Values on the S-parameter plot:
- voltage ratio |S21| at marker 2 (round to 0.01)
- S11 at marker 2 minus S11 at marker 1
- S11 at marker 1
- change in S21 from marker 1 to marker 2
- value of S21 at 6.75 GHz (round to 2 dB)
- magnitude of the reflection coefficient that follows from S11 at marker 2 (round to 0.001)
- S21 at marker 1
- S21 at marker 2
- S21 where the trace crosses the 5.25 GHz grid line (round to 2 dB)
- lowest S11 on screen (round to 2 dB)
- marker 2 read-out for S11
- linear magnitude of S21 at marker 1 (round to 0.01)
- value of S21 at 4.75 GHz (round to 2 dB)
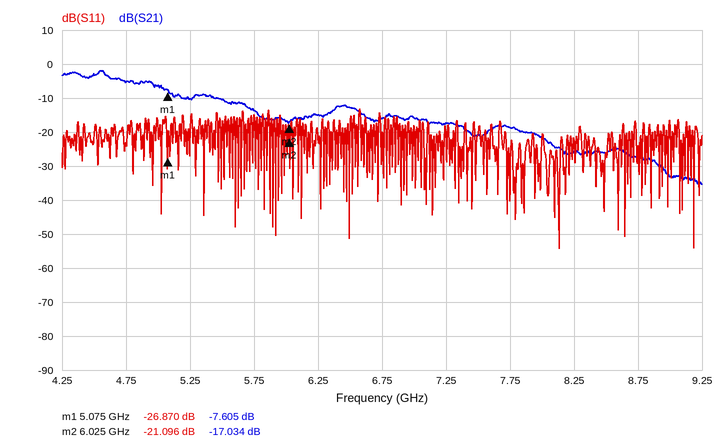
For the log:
0.14
5.774 dB
-26.870 dB
-9.429 dB
-16 dB
0.088
-7.605 dB
-17.034 dB
-10 dB
-54 dB
-21.096 dB
0.42
-6 dB
